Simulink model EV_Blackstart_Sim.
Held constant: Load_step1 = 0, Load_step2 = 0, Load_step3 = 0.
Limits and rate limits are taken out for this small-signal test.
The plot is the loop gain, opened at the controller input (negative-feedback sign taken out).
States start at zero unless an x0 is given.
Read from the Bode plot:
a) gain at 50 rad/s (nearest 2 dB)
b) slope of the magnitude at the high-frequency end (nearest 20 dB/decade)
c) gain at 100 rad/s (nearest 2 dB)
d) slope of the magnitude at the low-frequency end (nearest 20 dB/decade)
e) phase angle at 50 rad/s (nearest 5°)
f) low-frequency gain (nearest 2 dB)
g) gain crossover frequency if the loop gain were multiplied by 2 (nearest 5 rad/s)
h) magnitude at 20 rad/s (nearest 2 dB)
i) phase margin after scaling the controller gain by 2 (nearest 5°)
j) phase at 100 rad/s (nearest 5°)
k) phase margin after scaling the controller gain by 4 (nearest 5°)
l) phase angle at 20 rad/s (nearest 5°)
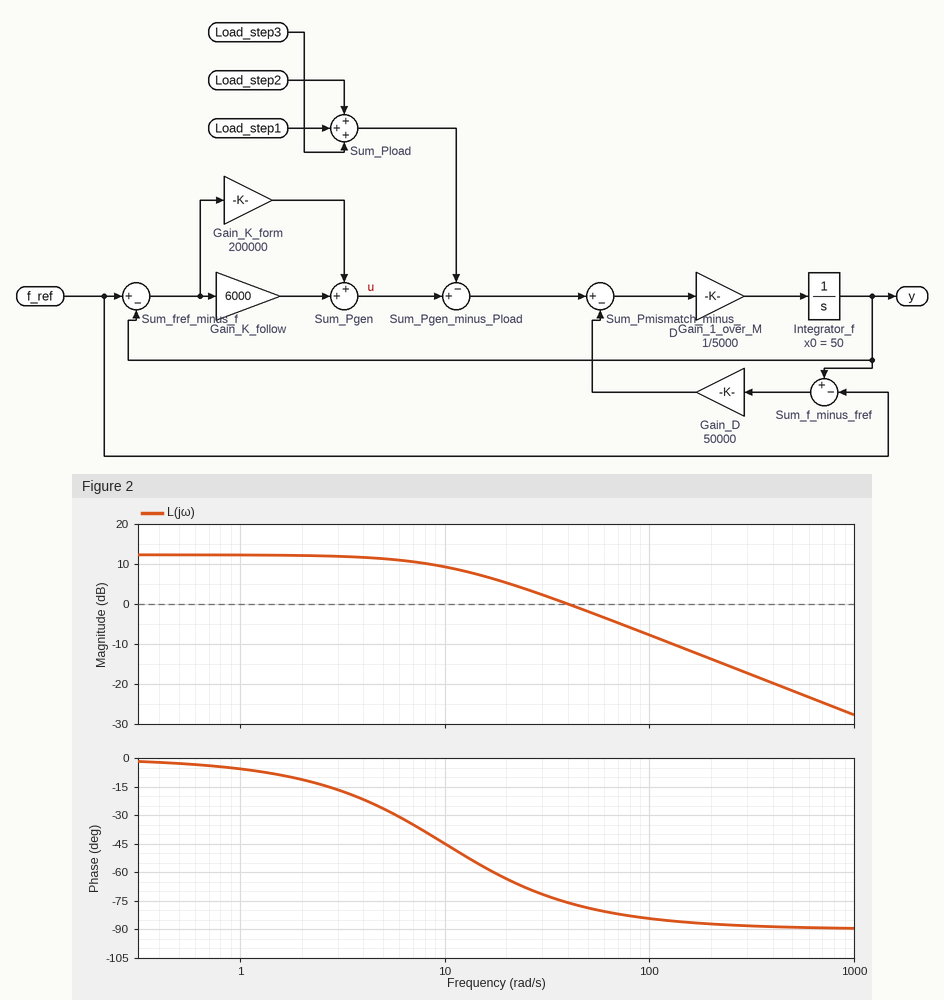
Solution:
-2 dB
-20 dB/decade
-8 dB
0 dB/decade
-80°
12 dB
80 rad/s
6 dB
95°
-85°
95°
-65°
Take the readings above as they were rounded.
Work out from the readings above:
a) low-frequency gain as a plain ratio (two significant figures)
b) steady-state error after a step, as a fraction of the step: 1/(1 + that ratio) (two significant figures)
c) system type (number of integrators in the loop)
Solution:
4.0
0.20
0
